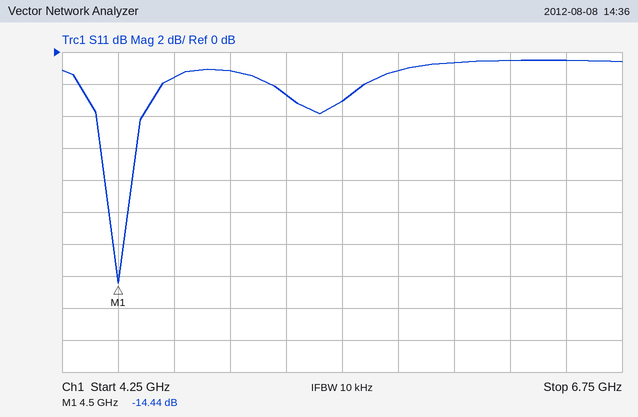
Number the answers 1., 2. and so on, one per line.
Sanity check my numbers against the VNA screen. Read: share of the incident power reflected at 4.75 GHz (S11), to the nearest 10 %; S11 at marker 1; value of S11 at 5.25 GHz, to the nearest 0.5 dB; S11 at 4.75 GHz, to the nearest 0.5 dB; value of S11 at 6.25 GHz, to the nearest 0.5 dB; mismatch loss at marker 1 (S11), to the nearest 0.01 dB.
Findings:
1. 70 %
2. -14.44 dB
3. -2.5 dB
4. -1.5 dB
5. -0.5 dB
6. 0.16 dB
